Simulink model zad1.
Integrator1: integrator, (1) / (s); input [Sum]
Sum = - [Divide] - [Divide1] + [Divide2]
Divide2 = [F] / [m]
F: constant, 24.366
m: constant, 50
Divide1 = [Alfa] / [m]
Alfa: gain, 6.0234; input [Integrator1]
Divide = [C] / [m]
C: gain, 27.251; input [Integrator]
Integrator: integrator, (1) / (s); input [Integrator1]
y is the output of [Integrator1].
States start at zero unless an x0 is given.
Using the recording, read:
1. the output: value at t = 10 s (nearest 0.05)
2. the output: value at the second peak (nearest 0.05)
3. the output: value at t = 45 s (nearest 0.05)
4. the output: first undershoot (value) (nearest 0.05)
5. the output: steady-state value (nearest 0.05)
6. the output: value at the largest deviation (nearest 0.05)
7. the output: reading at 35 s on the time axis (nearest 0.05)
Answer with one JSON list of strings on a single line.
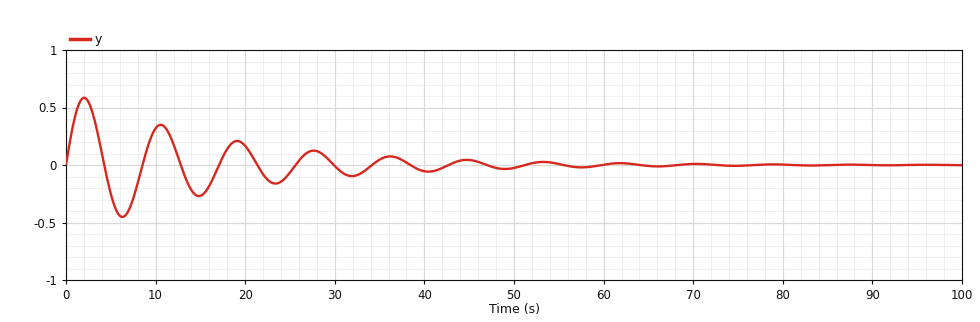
["0.30", "0.35", "0.05", "-0.45", "0.00", "0.60", "0.05"]
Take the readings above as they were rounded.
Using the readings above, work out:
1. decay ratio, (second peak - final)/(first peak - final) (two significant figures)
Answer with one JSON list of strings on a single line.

["0.58"]
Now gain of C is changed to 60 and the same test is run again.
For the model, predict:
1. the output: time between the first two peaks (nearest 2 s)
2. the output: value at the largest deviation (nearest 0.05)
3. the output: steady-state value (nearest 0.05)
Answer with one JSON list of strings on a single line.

["6 s", "0.40", "0.00"]
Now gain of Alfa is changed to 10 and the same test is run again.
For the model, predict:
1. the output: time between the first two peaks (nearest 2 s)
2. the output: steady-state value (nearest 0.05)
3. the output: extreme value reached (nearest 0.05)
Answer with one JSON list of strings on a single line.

["8 s", "0.00", "0.55"]
